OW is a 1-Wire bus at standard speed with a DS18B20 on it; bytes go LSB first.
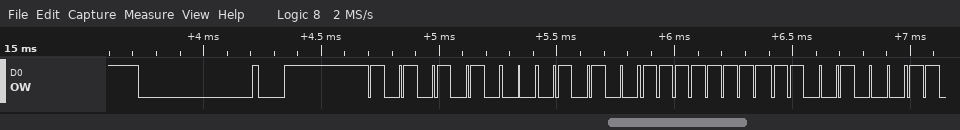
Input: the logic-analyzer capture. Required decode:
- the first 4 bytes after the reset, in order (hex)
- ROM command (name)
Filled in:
55 28 FF 13
Match ROM
